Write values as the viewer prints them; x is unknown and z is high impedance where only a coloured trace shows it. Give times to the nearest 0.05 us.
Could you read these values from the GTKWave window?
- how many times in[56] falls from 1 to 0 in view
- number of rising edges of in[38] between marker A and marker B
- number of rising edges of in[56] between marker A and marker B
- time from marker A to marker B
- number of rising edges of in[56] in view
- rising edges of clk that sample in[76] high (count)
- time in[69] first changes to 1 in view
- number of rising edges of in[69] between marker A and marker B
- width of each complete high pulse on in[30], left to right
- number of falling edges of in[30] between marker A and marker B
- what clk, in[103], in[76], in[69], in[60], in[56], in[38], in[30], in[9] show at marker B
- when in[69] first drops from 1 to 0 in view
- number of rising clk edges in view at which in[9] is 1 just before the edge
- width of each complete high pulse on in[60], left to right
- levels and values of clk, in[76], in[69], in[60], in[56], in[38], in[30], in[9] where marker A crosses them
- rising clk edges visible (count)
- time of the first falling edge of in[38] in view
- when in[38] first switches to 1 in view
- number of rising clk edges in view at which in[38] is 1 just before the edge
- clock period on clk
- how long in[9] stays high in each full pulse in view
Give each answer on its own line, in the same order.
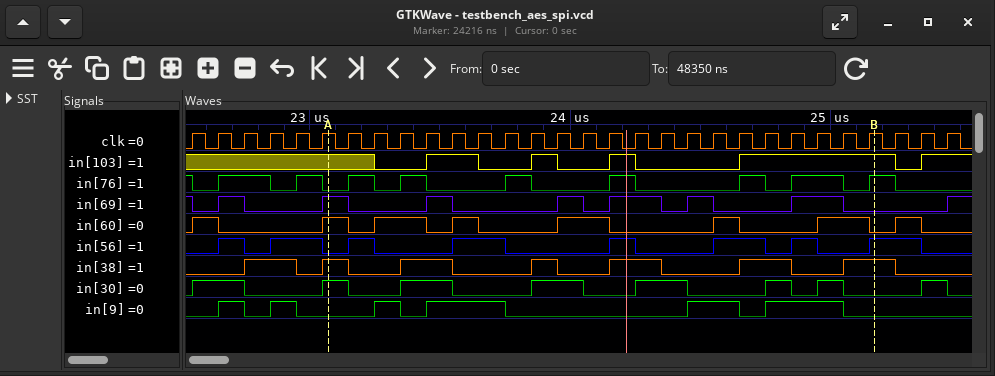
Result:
8
5
6
2.1 us
8
12
22.65 us
5
0.2 us, 0.1 us, 0.2 us, 0.2 us, 0.2 us, 0.1 us, 0.1 us, 0.1 us
6
clk=1, in[103]=1, in[76]=1, in[69]=0, in[60]=0, in[56]=1, in[38]=1, in[30]=0, in[9]=0
22.55 us
11
0.1 us, 0.1 us, 0.2 us, 0.1 us, 0.2 us, 0.1 us, 0.2 us, 0.1 us
clk=1, in[76]=0, in[69]=1, in[60]=1, in[56]=0, in[38]=1, in[30]=1, in[9]=0
30
22.95 us
22.75 us
12
0.1 us
0.1 us, 0.1 us, 0.1 us, 0.3 us, 0.2 us, 0.3 us
